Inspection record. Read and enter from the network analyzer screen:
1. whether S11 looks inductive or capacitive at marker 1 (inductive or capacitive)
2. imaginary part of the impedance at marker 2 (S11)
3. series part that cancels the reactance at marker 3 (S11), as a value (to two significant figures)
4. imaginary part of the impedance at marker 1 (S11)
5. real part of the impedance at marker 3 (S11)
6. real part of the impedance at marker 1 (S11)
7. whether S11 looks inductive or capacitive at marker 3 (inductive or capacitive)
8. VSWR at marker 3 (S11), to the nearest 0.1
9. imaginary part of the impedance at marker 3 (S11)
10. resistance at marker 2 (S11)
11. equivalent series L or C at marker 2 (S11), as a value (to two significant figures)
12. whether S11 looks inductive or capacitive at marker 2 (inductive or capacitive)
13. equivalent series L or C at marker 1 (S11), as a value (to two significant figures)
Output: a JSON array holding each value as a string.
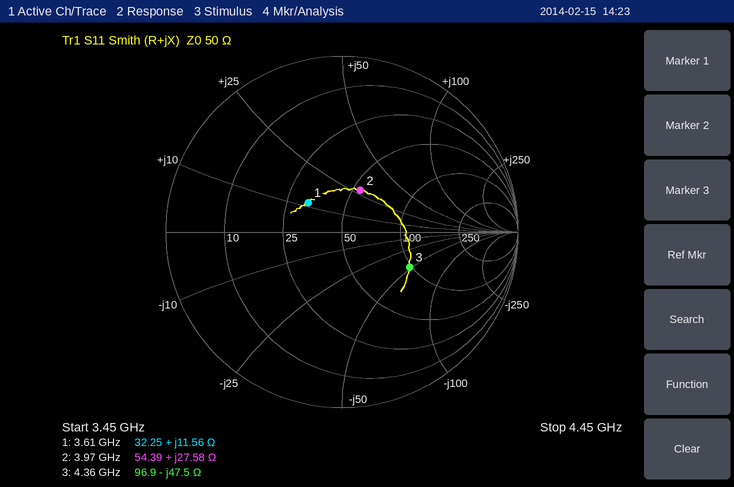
["inductive", "+27.58 Ω", "1.7 nH", "+11.56 Ω", "96.9 Ω", "32.25 Ω", "capacitive", "2.5", "-47.5 Ω", "54.39 Ω", "1.1 nH", "inductive", "510 pH"]
